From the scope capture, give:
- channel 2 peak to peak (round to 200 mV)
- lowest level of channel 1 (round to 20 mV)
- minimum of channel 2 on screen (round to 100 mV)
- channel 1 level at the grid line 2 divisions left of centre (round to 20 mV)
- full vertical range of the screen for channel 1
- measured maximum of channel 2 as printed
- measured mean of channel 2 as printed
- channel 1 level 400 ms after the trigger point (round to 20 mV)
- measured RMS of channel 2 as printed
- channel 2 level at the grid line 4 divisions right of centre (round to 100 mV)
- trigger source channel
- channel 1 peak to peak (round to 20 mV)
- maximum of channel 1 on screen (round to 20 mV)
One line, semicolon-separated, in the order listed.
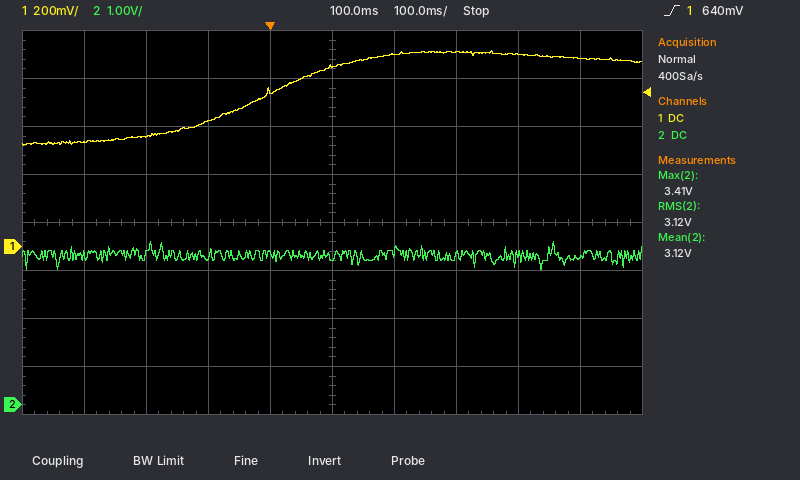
600 mV; 420 mV; 2.8 V; 520 mV; 1.6 V; 3.41 V; 3.12 V; 800 mV; 3.12 V; 3.1 V; channel 1; 400 mV; 820 mV
